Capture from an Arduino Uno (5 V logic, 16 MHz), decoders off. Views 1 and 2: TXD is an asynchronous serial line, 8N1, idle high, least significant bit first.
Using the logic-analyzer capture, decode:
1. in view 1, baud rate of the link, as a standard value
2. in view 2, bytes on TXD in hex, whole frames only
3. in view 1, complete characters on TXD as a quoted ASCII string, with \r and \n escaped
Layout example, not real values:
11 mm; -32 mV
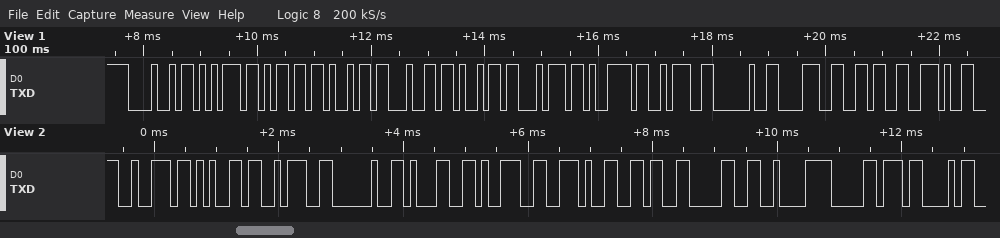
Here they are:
9600 baud; 72 65 3A 20 31 39 2E 36 30 C2 B0 43; "Humidity: 86."
